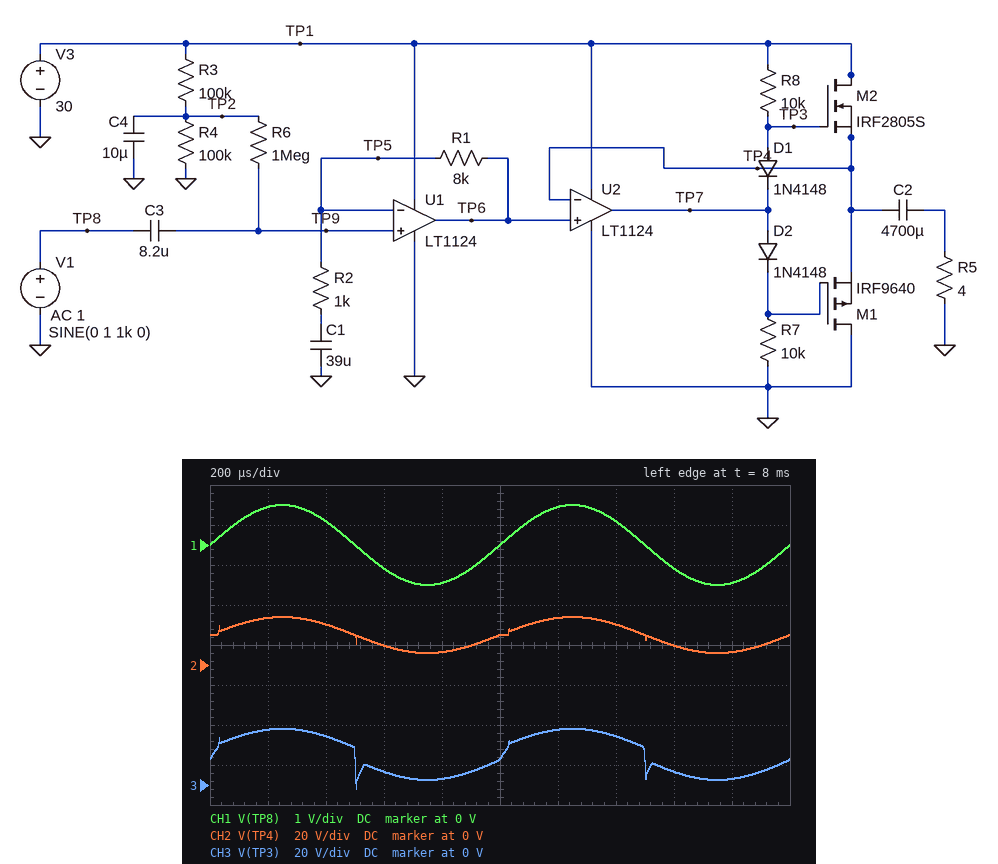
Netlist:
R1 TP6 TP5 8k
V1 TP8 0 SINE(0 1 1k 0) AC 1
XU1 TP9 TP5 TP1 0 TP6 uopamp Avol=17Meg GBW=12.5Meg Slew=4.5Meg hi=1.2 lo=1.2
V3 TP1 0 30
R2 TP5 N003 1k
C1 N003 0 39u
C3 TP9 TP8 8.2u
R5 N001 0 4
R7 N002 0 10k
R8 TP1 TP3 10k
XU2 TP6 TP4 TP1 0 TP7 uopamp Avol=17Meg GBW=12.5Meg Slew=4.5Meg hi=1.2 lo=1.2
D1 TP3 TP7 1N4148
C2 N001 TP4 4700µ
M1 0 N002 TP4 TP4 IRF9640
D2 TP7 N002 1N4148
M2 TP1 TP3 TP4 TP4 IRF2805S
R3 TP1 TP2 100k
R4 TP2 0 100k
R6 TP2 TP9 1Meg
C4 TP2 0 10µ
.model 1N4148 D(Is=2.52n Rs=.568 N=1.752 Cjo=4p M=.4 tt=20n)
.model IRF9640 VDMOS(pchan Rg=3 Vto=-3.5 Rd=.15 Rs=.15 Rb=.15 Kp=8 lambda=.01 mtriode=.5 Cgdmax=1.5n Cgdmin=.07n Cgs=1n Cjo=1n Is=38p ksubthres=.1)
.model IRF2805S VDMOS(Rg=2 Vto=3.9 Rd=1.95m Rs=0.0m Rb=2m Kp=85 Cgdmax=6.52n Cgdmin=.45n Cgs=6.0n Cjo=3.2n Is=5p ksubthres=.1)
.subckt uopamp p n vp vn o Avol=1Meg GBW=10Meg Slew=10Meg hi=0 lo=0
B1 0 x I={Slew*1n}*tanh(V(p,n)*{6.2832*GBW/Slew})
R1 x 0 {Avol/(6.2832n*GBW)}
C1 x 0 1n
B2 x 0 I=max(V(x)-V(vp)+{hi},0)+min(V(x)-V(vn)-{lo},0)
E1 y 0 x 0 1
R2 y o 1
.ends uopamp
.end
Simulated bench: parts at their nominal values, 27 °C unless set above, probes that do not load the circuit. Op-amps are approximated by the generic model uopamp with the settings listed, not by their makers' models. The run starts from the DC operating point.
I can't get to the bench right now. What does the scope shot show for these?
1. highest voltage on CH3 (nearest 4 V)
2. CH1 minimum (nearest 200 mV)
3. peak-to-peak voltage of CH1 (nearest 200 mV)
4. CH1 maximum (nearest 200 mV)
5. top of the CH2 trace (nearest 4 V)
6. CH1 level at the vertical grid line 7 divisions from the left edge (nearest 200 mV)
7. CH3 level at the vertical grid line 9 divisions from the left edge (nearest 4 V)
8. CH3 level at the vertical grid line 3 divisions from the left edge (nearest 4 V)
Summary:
28 V
-1.0 V
2.0 V
1.0 V
24 V
600 mV
4 V
8 V
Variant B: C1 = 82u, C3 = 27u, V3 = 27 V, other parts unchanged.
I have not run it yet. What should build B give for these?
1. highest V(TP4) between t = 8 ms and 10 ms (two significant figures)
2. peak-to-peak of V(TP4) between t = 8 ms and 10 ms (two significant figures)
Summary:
22 V
17 V
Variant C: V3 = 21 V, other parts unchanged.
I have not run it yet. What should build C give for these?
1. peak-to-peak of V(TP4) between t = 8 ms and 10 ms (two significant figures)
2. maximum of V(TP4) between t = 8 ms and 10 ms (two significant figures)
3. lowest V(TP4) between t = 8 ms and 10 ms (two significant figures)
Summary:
11 V
16 V
5.0 V
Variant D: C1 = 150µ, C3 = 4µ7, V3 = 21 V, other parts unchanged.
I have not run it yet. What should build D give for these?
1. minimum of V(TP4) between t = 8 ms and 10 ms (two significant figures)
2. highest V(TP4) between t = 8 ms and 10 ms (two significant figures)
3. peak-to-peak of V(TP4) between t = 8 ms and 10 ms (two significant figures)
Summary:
5.0 V
16 V
11 V
